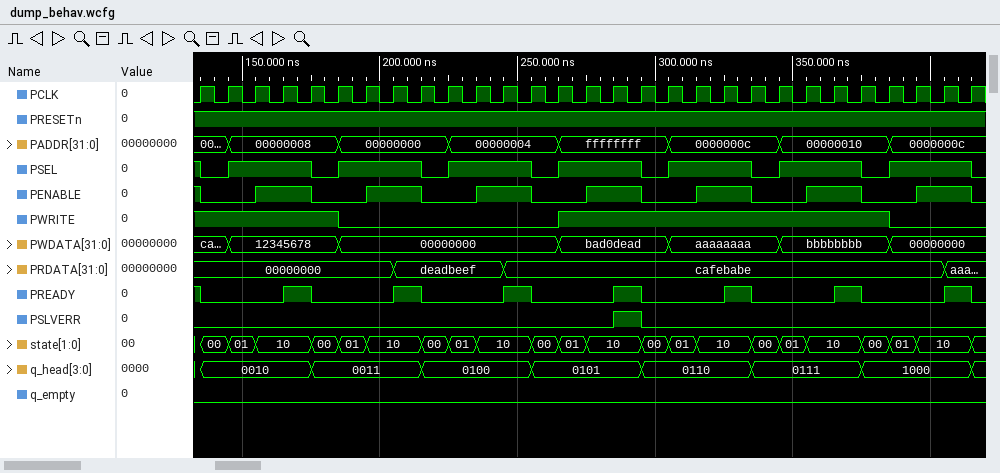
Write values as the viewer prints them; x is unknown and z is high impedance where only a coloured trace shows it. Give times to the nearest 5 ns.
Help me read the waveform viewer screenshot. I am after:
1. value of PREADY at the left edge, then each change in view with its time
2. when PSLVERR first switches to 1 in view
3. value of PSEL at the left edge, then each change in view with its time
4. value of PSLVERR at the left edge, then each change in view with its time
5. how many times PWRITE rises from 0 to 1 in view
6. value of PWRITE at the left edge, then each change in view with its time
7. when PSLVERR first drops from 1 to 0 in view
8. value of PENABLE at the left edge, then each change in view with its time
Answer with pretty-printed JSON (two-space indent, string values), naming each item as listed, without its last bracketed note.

{
  "value of PREADY at the left edge, then each change in view with its time": "1, 0 at 135 ns, 1 at 165 ns, 0 at 175 ns, 1 at 205 ns, 0 at 215 ns, 1 at 245 ns, 0 at 255 ns, 1 at 285 ns, 0 at 295 ns, 1 at 325 ns, 0 at 335 ns, 1 at 365 ns, 0 at 375 ns, 1 at 405 ns, 0 at 415 ns",
  "when PSLVERR first switches to 1 in view": "285 ns",
  "value of PSEL at the left edge, then each change in view with its time": "1, 0 at 135 ns, 1 at 145 ns, 0 at 175 ns, 1 at 185 ns, 0 at 215 ns, 1 at 225 ns, 0 at 255 ns, 1 at 265 ns, 0 at 295 ns, 1 at 305 ns, 0 at 335 ns, 1 at 345 ns, 0 at 375 ns, 1 at 385 ns, 0 at 415 ns",
  "value of PSLVERR at the left edge, then each change in view with its time": "0, 1 at 285 ns, 0 at 295 ns",
  "how many times PWRITE rises from 0 to 1 in view": "1",
  "value of PWRITE at the left edge, then each change in view with its time": "1, 0 at 185 ns, 1 at 265 ns, 0 at 385 ns",
  "when PSLVERR first drops from 1 to 0 in view": "295 ns",
  "value of PENABLE at the left edge, then each change in view with its time": "1, 0 at 135 ns, 1 at 155 ns, 0 at 175 ns, 1 at 195 ns, 0 at 215 ns, 1 at 235 ns, 0 at 255 ns, 1 at 275 ns, 0 at 295 ns, 1 at 315 ns, 0 at 335 ns, 1 at 355 ns, 0 at 375 ns, 1 at 395 ns, 0 at 415 ns"
}
